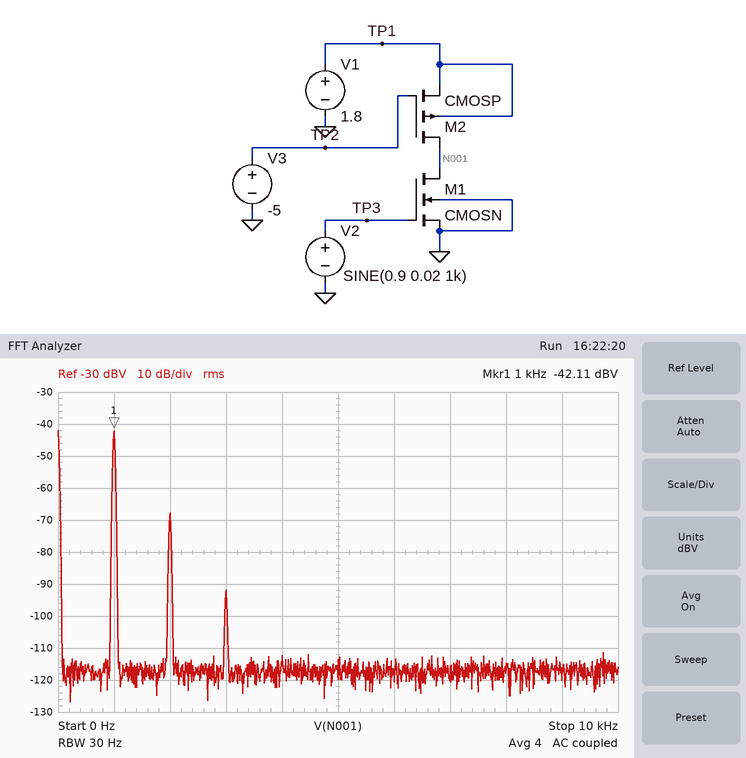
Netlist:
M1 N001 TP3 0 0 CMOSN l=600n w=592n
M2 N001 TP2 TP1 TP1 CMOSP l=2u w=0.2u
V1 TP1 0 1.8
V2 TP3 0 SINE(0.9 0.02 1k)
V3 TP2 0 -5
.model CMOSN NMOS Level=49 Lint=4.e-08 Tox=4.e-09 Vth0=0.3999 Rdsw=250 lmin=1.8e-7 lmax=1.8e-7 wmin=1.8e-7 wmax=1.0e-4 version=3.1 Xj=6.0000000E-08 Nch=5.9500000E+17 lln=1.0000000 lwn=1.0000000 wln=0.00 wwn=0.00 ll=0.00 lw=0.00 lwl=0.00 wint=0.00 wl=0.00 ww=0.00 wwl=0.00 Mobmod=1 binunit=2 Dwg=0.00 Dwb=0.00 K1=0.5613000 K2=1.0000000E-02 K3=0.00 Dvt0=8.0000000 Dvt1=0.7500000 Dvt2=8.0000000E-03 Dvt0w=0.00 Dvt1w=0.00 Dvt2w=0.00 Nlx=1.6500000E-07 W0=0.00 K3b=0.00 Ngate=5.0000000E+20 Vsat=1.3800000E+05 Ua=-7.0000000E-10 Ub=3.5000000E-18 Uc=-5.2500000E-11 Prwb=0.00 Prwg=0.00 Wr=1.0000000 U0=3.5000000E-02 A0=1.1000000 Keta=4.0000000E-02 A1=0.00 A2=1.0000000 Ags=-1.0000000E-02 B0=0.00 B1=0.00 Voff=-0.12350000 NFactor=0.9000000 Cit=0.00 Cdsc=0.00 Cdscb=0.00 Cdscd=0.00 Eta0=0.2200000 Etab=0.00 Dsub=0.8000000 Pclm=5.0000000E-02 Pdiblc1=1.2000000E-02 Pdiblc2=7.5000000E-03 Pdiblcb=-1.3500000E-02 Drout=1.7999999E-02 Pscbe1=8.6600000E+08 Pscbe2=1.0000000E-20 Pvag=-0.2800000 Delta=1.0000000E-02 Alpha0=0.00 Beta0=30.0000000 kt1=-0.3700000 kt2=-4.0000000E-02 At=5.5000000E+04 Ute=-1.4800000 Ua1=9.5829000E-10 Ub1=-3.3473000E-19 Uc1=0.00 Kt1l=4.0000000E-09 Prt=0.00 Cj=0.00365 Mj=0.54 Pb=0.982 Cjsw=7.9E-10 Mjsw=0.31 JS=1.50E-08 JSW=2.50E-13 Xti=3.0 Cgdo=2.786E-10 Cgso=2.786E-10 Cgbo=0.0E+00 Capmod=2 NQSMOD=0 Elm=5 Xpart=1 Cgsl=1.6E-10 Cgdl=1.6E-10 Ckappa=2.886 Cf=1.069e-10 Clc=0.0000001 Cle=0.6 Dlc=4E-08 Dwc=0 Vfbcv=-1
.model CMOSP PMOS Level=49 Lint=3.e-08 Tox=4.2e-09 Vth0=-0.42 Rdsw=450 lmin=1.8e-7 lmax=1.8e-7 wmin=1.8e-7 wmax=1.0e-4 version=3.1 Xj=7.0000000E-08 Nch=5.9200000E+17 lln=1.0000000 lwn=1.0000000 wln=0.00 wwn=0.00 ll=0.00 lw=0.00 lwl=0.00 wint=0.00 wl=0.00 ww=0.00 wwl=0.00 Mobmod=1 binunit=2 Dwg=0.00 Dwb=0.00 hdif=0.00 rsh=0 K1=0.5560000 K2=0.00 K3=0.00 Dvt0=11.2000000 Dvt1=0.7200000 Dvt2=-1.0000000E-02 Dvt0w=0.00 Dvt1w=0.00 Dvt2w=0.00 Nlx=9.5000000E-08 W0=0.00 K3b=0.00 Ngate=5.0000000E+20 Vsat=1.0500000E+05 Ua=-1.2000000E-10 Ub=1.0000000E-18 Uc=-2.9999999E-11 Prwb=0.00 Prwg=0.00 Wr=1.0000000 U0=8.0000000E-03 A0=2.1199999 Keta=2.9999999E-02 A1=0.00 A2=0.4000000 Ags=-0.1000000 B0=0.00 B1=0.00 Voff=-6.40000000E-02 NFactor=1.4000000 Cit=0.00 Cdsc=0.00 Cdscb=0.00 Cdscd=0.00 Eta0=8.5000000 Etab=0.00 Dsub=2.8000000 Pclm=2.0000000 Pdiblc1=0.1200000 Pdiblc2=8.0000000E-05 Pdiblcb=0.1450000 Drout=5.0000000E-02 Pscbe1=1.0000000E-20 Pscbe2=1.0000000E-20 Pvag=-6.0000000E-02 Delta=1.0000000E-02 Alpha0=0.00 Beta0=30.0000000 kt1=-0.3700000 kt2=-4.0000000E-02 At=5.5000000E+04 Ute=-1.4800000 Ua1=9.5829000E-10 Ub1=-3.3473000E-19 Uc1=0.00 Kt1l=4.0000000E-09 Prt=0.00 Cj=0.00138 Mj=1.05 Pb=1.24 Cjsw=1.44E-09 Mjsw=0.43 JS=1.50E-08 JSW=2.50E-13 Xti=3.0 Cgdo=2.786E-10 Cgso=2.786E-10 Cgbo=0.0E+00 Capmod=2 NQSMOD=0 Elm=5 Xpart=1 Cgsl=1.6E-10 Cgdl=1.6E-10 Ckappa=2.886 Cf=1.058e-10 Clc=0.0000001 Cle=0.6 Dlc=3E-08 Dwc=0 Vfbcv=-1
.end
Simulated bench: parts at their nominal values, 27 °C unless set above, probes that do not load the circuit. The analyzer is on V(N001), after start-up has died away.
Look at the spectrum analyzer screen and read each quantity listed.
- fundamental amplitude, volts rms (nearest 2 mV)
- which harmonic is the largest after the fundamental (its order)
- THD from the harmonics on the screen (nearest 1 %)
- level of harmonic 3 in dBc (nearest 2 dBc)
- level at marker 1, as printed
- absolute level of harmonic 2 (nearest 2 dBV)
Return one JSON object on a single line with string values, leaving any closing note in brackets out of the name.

{"fundamental amplitude, volts rms": "8 mV", "which harmonic is the largest after the fundamental": "2", "THD from the harmonics on the screen": "5 %", "level of harmonic 3 in dBc": "-50 dBc", "level at marker 1, as printed": "-42.11 dBV", "absolute level of harmonic 2": "-68 dBV"}
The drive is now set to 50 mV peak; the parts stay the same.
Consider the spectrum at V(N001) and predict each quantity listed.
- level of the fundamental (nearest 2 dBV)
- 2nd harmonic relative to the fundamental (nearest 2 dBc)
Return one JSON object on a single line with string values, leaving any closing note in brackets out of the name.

{"level of the fundamental": "-34 dBV", "2nd harmonic relative to the fundamental": "-18 dBc"}
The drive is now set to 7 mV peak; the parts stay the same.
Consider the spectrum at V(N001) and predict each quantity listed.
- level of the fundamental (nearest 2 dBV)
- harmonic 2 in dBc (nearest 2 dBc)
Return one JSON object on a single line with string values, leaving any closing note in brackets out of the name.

{"level of the fundamental": "-52 dBV", "harmonic 2 in dBc": "-34 dBc"}
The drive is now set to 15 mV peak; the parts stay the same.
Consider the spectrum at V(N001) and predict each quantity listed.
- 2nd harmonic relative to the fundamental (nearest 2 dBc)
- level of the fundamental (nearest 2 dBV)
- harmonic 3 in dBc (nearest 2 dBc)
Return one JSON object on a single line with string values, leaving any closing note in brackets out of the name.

{"2nd harmonic relative to the fundamental": "-28 dBc", "level of the fundamental": "-44 dBV", "harmonic 3 in dBc": "-54 dBc"}
